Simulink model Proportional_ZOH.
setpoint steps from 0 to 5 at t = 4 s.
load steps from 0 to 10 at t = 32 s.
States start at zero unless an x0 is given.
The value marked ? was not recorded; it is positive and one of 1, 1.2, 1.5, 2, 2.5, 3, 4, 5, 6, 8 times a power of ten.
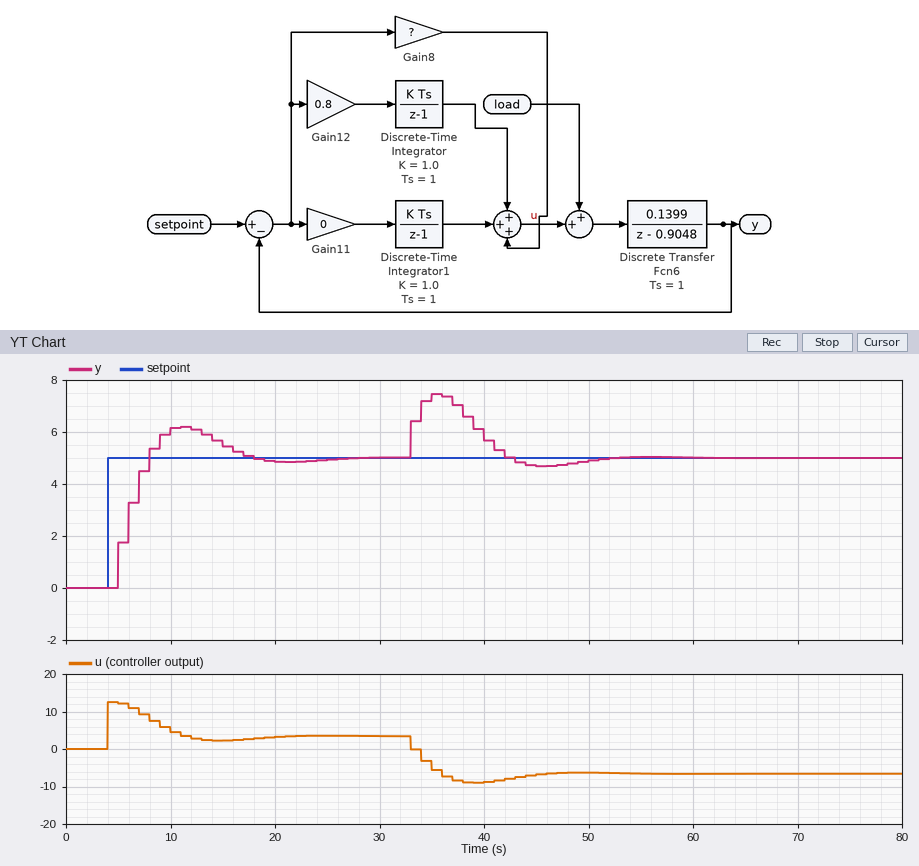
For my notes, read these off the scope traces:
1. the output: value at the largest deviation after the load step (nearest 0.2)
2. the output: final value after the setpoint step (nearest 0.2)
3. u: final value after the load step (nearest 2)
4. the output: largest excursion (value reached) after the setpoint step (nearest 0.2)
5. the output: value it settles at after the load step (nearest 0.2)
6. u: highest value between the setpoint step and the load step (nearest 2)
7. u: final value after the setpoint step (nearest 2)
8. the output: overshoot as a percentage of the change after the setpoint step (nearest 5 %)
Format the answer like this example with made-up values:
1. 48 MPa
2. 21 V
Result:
1. 7.4
2. 5.0
3. -6
4. 6.2
5. 5.0
6. 12
7. 4
8. 25 %
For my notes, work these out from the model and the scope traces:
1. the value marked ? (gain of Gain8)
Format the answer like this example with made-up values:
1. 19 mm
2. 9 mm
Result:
1. 2.5
